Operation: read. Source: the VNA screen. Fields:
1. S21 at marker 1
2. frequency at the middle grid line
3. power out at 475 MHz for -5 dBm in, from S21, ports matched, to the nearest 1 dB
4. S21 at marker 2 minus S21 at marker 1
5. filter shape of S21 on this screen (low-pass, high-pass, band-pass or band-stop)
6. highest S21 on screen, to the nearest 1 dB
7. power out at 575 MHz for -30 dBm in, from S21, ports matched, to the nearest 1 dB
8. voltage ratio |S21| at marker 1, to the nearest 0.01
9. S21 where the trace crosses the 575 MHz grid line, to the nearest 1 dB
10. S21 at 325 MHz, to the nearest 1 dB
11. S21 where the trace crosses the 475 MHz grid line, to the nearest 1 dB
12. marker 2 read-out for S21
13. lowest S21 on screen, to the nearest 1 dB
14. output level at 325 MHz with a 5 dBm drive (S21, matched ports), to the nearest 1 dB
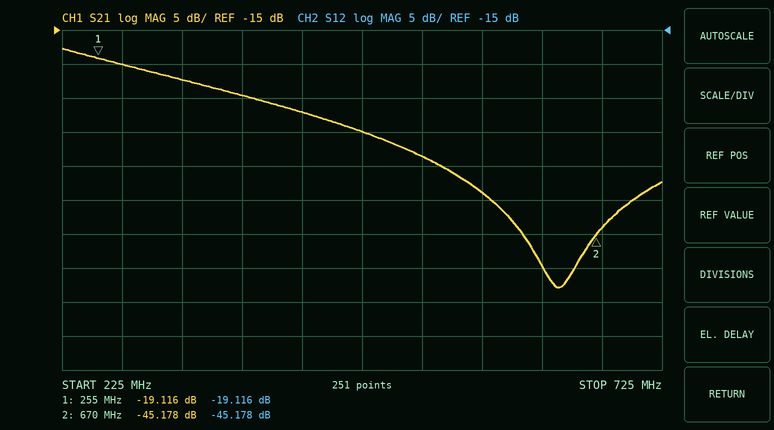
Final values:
-19.116 dB
475 MHz
-35 dBm
-26.062 dB
low-pass
-18 dB
-69 dBm
0.11
-39 dB
-22 dB
-30 dB
-45.178 dB
-53 dB
-17 dBm
